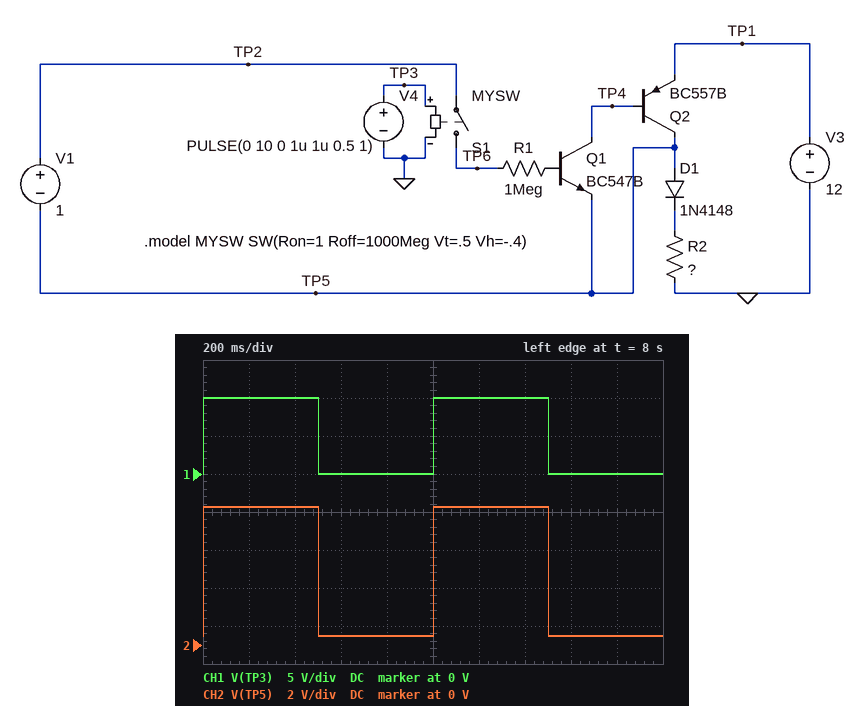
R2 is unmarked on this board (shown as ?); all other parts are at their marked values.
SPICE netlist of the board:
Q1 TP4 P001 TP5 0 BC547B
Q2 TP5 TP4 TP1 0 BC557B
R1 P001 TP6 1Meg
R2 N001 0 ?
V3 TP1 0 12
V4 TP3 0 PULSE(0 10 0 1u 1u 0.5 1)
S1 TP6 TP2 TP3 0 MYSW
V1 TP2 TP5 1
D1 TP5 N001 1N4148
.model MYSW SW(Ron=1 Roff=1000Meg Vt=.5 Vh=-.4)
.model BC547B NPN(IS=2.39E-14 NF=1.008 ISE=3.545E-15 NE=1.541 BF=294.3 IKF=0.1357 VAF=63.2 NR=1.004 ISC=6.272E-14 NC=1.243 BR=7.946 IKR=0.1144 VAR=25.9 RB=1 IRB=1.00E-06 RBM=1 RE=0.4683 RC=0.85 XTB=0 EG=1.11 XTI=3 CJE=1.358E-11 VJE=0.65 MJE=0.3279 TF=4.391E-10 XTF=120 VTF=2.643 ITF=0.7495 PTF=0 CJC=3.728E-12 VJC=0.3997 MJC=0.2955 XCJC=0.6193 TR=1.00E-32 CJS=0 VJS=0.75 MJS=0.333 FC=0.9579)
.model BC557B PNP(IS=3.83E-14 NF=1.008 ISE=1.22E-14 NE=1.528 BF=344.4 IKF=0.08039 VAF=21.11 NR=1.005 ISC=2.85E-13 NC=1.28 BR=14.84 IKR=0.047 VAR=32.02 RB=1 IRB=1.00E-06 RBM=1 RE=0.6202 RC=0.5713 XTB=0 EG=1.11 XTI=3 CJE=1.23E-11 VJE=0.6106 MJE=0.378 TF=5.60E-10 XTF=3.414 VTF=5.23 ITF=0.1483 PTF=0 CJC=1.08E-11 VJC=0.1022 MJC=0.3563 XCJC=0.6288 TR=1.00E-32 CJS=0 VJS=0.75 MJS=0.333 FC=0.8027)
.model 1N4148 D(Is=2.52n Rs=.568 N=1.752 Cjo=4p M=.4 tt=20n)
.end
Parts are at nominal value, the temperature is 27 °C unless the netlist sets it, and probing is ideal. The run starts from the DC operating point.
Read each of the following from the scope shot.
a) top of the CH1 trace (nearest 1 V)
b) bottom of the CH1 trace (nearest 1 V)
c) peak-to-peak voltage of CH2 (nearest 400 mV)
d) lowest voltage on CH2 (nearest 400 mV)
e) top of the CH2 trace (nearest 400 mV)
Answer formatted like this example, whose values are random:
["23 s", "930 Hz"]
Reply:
["10 V", "0 V", "6.8 V", "400 mV", "7.2 V"]
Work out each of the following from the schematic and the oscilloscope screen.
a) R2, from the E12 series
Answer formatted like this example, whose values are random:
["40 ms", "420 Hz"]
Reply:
["180 Ω"]
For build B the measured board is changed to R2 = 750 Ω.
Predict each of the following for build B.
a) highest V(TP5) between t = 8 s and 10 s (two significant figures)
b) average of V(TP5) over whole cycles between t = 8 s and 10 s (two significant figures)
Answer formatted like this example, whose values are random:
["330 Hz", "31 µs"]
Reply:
["11 V", "5.9 V"]
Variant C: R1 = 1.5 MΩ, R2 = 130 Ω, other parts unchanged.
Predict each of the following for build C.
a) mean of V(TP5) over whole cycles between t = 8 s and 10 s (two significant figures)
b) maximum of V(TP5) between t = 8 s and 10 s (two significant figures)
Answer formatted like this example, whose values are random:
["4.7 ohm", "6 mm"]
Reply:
["2.6 V", "4.7 V"]
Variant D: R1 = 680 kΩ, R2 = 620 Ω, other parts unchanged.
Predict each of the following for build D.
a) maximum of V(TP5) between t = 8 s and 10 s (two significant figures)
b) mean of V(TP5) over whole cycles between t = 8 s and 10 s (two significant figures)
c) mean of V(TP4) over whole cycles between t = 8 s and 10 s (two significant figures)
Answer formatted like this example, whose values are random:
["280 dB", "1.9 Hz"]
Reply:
["11 V", "5.9 V", "11 V"]
